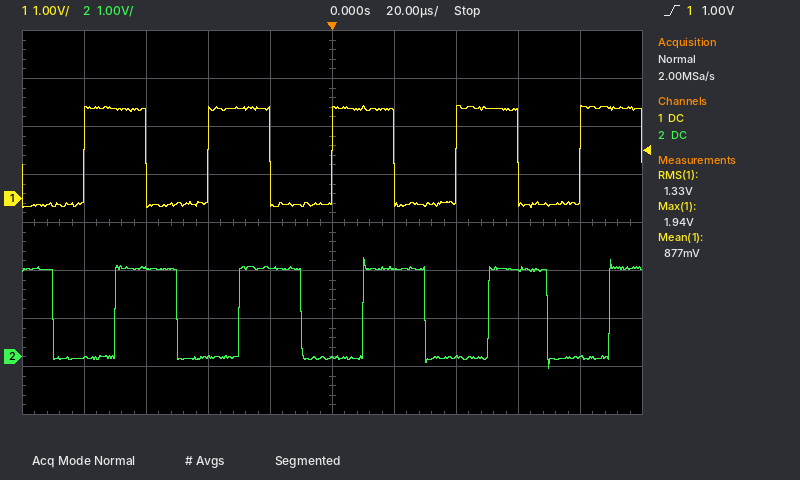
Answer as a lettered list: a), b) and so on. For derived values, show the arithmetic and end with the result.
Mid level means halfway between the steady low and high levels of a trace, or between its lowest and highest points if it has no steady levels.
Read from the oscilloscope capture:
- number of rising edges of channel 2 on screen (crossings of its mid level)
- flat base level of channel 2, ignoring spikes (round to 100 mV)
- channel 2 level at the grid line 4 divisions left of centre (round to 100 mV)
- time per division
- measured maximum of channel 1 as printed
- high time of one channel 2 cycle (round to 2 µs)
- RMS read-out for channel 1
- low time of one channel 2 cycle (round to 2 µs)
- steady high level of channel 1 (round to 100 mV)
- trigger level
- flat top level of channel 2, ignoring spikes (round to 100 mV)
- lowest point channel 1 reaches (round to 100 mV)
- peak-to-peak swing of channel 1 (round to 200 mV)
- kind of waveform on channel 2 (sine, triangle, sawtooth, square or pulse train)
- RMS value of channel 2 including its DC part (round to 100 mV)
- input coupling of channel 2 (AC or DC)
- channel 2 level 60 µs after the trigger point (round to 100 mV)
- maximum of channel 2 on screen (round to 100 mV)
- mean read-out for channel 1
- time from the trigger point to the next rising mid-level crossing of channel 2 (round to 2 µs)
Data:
a) 5
b) 0.0 V
c) 0.0 V
d) 20 µs
e) 1.94 V
f) 20 µs
g) 1.33 V
h) 20 µs
i) 1.9 V
j) 1.00 V
k) 1.8 V
l) -200 mV
m) 2.2 V
n) square
o) √(0.5 × (1.8 V)² + 0.5 × (0.0 V)²) ≈ 1.3 V
p) DC
q) 1.8 V
r) 2.1 V
s) 877 mV
t) 10 µs
